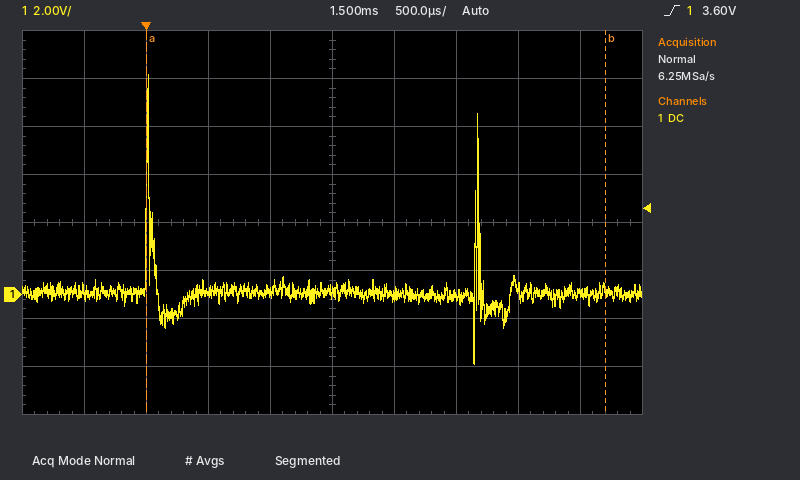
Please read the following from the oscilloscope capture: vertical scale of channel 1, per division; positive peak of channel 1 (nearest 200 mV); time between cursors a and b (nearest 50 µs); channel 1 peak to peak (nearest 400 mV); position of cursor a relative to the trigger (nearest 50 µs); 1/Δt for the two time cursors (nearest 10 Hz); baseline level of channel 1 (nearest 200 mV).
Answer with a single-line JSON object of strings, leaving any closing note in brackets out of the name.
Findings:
{"vertical scale of channel 1, per division": "2 V", "positive peak of channel 1": "9.2 V", "time between cursors a and b": "3.70 ms", "channel 1 peak to peak": "12.0 V", "position of cursor a relative to the trigger": "0 µs", "1/Δt for the two time cursors": "270 Hz", "baseline level of channel 1": "0.0 V"}
